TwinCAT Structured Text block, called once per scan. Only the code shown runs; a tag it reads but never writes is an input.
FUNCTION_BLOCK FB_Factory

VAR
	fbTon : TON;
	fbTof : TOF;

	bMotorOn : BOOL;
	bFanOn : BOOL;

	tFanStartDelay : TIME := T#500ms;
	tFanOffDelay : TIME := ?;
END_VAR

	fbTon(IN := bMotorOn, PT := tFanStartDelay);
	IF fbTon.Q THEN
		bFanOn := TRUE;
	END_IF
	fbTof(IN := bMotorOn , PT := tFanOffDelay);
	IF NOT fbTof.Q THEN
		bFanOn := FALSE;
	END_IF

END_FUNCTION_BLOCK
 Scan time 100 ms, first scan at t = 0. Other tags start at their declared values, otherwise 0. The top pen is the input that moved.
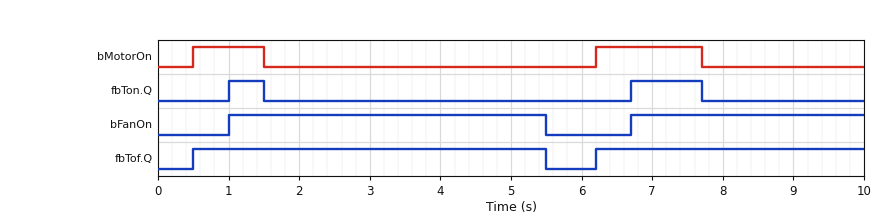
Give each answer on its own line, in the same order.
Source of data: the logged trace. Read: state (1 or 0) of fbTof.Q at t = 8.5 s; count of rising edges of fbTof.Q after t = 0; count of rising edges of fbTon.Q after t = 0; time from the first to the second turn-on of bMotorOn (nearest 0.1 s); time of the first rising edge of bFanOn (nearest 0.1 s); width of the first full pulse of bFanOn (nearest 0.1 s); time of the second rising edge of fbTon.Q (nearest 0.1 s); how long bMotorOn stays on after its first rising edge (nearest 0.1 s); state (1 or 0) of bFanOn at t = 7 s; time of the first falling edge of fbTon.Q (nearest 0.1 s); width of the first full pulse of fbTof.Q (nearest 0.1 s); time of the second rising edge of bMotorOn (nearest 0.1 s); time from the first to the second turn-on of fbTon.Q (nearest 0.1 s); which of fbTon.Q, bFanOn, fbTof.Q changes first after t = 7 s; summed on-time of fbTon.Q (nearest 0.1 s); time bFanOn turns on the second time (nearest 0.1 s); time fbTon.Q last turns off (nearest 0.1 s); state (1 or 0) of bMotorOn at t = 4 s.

1
2
2
5.7 s
1.0 s
4.5 s
6.7 s
1.0 s
1
1.5 s
5.0 s
6.2 s
5.7 s
fbTon.Q
1.5 s
6.7 s
7.7 s
0
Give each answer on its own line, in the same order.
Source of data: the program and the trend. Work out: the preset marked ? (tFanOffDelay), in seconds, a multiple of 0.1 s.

4.0 s
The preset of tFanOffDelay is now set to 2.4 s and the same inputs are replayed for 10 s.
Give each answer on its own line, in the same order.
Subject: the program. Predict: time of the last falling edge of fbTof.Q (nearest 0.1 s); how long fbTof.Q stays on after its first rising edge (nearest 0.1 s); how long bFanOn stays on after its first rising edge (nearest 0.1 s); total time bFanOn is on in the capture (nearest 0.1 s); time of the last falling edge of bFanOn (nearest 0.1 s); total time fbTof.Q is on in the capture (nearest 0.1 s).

3.9 s
3.4 s
2.9 s
6.2 s
3.9 s
7.2 s
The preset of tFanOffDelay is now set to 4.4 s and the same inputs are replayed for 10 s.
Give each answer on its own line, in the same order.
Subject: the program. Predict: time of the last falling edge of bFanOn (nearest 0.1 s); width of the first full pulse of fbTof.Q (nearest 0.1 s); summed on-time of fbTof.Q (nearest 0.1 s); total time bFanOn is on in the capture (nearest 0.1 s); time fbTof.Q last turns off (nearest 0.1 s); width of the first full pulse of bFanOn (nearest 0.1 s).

5.9 s
5.4 s
9.2 s
8.2 s
5.9 s
4.9 s
